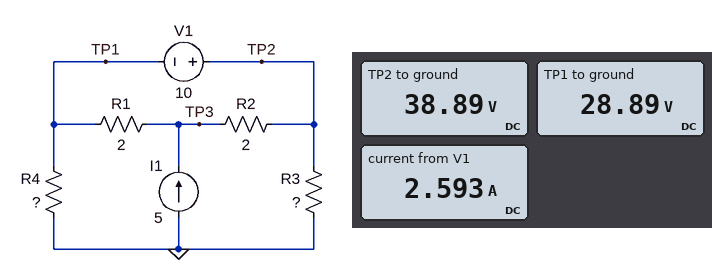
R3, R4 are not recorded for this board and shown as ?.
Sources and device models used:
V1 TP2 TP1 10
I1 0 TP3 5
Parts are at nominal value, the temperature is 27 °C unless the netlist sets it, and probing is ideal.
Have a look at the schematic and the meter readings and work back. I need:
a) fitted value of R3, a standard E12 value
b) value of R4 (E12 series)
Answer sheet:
15 Ω
12 Ω
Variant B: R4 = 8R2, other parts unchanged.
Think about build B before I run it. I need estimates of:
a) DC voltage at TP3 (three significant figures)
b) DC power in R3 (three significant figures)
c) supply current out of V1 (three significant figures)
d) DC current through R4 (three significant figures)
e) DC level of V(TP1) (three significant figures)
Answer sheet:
33.0 V
72.5 W
2.20 A
2.80 A
23.0 V
